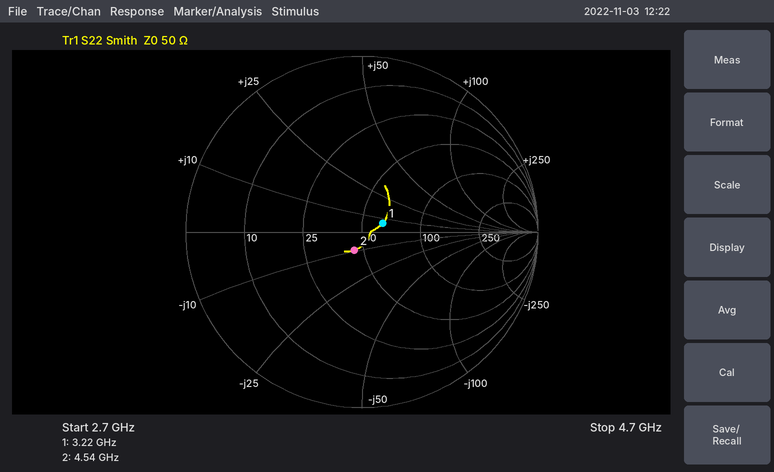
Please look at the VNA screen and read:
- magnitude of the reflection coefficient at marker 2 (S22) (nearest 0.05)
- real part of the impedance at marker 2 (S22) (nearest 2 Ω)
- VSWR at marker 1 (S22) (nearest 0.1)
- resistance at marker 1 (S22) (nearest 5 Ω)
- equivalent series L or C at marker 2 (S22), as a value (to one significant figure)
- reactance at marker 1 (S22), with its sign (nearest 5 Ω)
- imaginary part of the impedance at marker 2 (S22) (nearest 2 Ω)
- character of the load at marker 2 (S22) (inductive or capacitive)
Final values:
0.10
44 Ω
1.3
65 Ω
4 pF
+5 Ω
-10 Ω
capacitive
